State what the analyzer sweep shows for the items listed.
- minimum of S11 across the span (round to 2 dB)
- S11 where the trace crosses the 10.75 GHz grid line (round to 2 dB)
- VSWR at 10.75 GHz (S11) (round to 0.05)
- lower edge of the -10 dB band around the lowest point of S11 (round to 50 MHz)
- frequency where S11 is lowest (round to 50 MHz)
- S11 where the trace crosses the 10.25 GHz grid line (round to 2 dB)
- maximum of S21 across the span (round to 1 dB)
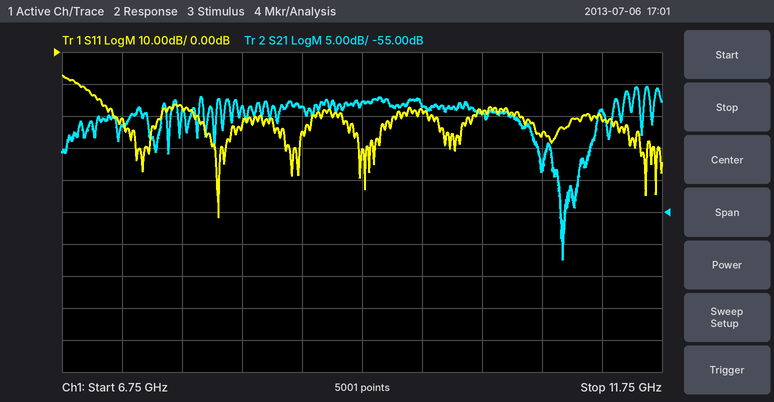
-52 dB
-26 dB
1.10
6.90 GHz
8.05 GHz
-20 dB
-35 dB
